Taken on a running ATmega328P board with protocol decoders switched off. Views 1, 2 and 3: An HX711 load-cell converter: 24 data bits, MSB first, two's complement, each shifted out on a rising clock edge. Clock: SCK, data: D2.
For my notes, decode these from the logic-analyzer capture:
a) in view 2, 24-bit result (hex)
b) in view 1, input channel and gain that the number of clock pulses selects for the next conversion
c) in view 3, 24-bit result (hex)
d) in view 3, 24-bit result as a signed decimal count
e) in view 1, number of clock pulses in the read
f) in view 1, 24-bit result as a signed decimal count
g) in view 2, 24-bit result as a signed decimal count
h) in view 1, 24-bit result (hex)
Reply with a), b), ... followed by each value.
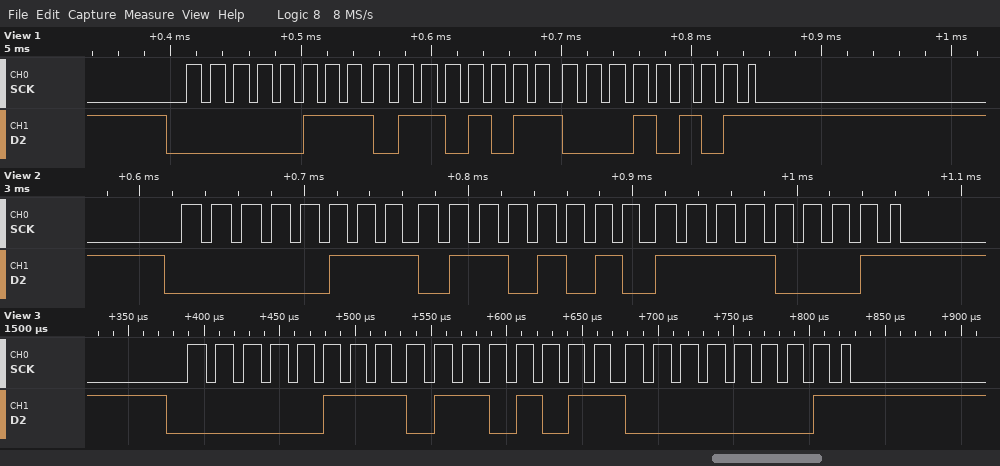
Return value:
a) 0x076AF1
b) channel A, gain 128
c) 0x076B01
d) 486145
e) 25
f) 486165
g) 486129
h) 0x076B15
